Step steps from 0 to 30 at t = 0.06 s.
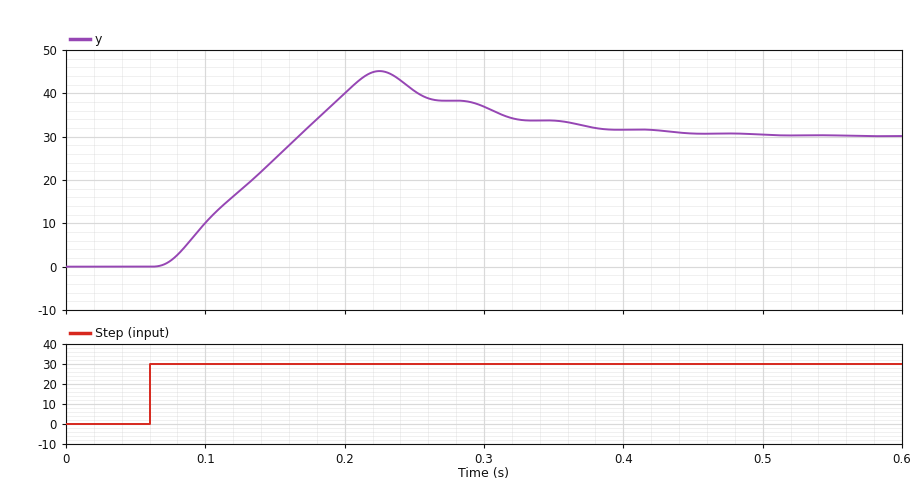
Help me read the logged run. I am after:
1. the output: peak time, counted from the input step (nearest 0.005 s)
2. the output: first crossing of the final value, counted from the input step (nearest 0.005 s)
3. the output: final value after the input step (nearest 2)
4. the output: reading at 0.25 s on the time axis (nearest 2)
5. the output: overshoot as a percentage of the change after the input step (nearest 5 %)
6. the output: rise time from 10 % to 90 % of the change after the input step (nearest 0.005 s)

0.165 s
0.105 s
30
40
50 %
0.075 s
